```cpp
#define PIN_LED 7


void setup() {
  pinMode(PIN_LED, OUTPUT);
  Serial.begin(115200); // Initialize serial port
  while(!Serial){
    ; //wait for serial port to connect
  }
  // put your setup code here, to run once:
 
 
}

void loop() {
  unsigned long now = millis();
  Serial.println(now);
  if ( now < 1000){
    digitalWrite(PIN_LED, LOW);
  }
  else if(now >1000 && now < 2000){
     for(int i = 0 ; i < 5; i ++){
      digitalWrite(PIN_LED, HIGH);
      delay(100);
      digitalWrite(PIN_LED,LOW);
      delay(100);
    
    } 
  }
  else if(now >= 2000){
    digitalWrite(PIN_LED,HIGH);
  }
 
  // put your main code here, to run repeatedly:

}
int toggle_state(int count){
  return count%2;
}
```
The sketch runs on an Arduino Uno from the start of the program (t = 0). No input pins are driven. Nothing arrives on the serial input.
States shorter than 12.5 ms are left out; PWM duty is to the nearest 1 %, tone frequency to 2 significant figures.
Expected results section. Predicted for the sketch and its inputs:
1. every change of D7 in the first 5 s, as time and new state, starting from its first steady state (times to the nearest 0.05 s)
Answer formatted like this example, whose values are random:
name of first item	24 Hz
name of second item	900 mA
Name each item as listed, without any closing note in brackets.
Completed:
every change of D7 in the first 5 s, as time and new state, starting from its first steady state	0 s low; 1 s high; 1.1 s low; 1.2 s high; 1.3 s low; 1.4 s high; 1.5 s low; 1.6 s high; 1.7 s low; 1.8 s high; 1.9 s low; 2 s high
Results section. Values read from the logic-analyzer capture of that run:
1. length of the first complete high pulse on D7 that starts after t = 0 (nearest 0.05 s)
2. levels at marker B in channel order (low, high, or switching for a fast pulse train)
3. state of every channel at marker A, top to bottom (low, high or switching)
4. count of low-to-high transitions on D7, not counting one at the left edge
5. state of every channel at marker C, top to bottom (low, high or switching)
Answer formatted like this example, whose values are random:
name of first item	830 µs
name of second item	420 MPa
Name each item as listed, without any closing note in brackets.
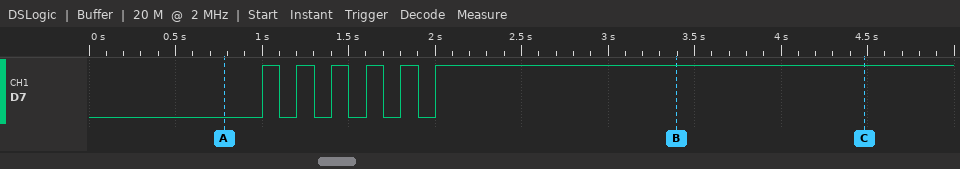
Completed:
length of the first complete high pulse on D7 that starts after t = 0	0.10 s
levels at marker B in channel order	D7 high
state of every channel at marker A, top to bottom	D7 low
count of low-to-high transitions on D7, not counting one at the left edge	6
state of every channel at marker C, top to bottom	D7 high
